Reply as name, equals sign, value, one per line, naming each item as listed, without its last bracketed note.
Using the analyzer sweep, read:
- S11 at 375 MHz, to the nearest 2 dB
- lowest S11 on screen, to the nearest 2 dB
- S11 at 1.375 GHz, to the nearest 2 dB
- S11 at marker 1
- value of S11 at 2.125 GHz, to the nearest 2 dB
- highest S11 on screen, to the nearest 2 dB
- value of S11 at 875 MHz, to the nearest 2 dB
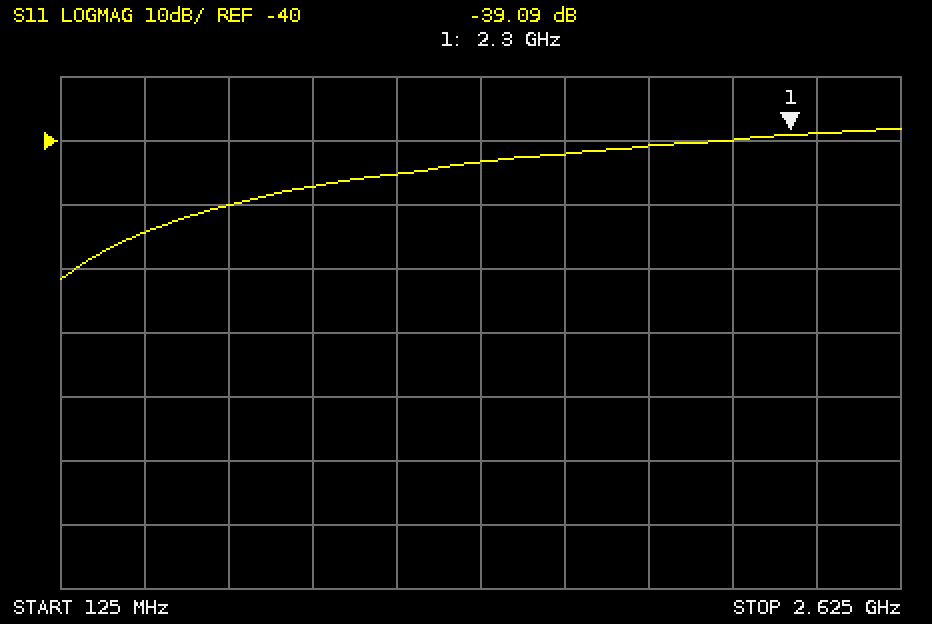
S11 at 375 MHz, to the nearest 2 dB = -54 dB
lowest S11 on screen, to the nearest 2 dB = -62 dB
S11 at 1.375 GHz, to the nearest 2 dB = -44 dB
S11 at marker 1 = -39.09 dB
value of S11 at 2.125 GHz, to the nearest 2 dB = -40 dB
highest S11 on screen, to the nearest 2 dB = -38 dB
value of S11 at 875 MHz, to the nearest 2 dB = -48 dB
